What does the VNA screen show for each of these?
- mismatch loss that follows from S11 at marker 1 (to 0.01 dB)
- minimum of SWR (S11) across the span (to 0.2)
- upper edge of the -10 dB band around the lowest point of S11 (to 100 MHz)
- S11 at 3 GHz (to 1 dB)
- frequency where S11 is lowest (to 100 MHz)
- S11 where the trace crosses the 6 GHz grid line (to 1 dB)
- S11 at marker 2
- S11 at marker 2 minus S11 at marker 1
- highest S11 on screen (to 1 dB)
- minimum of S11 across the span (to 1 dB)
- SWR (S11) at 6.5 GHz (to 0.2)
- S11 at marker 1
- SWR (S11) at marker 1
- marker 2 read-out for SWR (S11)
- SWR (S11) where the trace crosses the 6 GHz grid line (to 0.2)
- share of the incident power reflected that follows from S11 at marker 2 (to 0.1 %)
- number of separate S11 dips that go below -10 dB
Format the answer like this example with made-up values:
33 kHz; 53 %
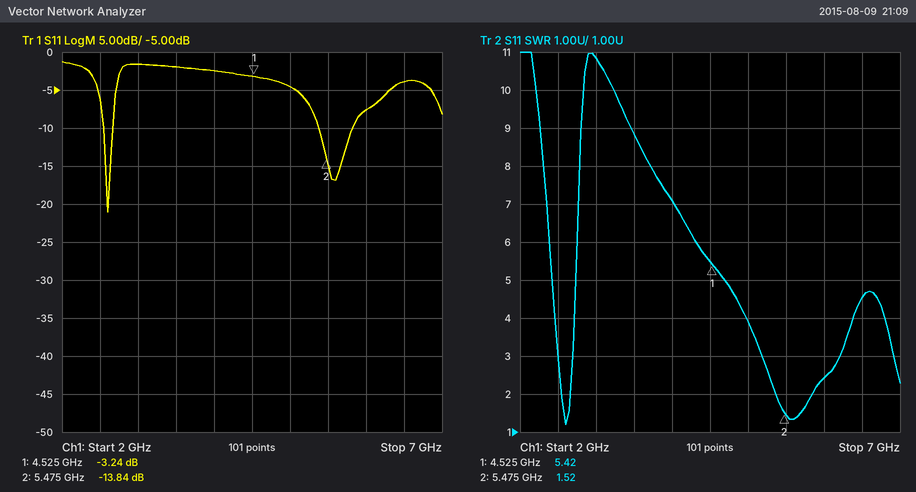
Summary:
2.79 dB; 1.2; 2.7 GHz; -2 dB; 2.6 GHz; -8 dB; -13.84 dB; -10.60 dB; -1 dB; -21 dB; 4.6; -3.24 dB; 5.42; 1.52; 2.4; 4.1 %; 2
